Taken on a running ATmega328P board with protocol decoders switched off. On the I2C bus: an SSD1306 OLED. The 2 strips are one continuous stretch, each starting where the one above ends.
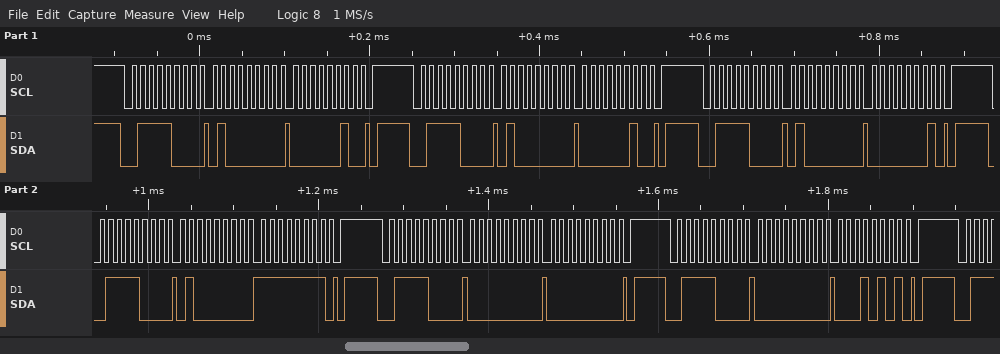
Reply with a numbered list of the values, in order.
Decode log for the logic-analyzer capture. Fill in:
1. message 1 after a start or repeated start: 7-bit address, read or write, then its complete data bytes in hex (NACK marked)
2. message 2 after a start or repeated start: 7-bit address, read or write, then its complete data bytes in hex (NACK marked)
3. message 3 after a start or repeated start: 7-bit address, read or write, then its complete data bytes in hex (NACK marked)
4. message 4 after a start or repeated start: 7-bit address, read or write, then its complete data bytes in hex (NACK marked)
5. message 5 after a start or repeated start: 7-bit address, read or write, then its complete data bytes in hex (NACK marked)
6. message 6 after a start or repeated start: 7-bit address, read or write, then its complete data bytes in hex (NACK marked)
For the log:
1. 0x3C write: 40 02
2. 0x3C write: 40 02
3. 0x3C write: 40 01
4. 0x3C write: 40 FF
5. 0x3C write: 00 00
6. 0x3C write: 00 15
